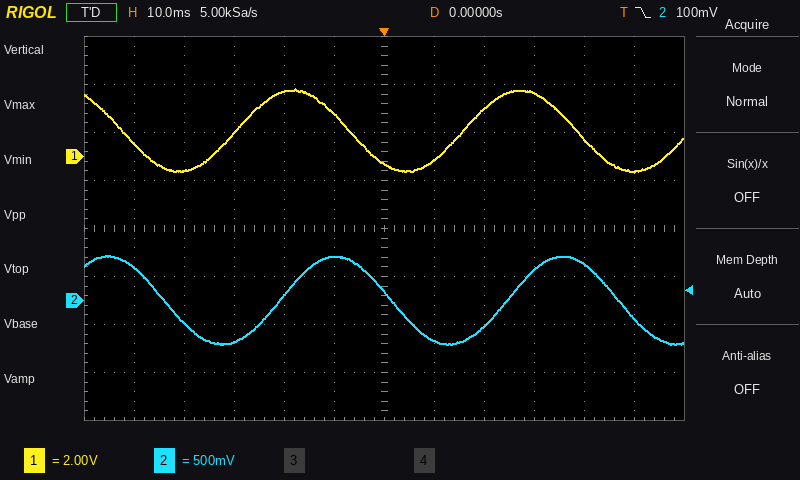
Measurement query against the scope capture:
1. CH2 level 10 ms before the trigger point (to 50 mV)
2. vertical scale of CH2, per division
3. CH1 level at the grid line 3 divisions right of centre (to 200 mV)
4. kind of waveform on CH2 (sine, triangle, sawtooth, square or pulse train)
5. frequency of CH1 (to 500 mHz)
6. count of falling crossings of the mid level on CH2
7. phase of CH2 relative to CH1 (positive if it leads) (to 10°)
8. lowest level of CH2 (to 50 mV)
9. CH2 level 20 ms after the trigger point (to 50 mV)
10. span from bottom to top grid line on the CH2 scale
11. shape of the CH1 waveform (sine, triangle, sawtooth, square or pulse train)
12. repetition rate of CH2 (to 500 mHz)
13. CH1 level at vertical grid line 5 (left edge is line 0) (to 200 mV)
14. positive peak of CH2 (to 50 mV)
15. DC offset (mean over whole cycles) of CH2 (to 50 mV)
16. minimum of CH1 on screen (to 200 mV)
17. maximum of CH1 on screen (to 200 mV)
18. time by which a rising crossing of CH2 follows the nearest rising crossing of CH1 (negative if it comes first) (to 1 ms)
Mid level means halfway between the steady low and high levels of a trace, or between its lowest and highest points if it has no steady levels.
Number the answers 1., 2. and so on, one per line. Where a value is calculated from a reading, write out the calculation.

1. 450 mV
2. 500 mV
3. 2.6 V
4. sine
5. 22.0 Hz
6. 3
7. -70°
8. -450 mV
9. -250 mV
10. 4 V
11. sine
12. 22.0 Hz
13. 1.8 V
14. 450 mV
15. (450 mV + (-450 mV)) / 2 ≈ 0 mV
16. -600 mV
17. 2.8 V
18. +9 ms
